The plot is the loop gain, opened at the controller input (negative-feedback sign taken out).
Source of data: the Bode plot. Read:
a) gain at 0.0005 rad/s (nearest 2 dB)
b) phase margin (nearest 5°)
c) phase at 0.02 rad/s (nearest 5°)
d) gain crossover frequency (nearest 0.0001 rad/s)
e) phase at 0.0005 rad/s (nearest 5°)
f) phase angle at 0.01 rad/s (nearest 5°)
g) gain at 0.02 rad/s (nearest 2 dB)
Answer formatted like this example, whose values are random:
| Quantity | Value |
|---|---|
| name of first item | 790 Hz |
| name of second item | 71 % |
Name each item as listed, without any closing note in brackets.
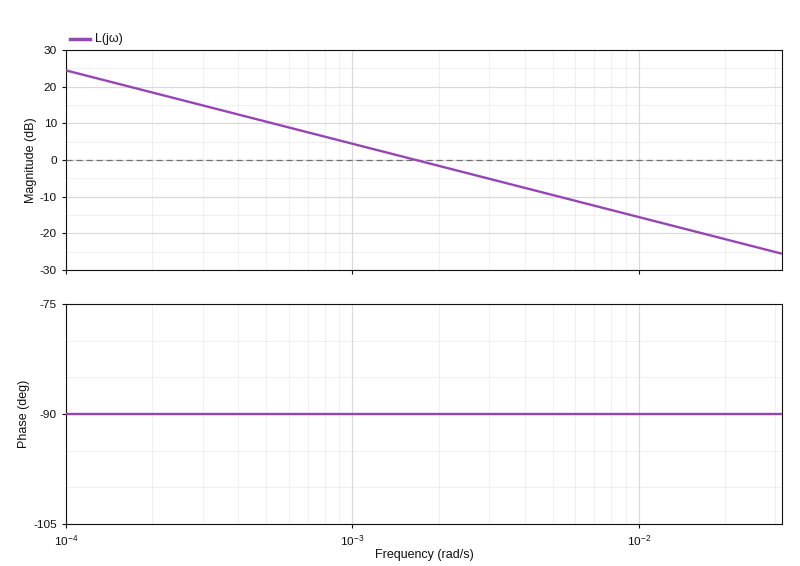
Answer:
| Quantity | Value |
|---|---|
| gain at 0.0005 rad/s | 10 dB |
| phase margin | 90° |
| phase at 0.02 rad/s | -90° |
| gain crossover frequency | 0.0017 rad/s |
| phase at 0.0005 rad/s | -90° |
| phase angle at 0.01 rad/s | -90° |
| gain at 0.02 rad/s | -22 dB |
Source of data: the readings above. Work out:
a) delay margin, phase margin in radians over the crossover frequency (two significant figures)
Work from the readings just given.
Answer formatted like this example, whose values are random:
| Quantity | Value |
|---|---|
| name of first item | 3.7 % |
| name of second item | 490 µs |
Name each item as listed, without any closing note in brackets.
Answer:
| Quantity | Value |
|---|---|
| delay margin, phase margin in radians over the crossover frequency | 920 s |
